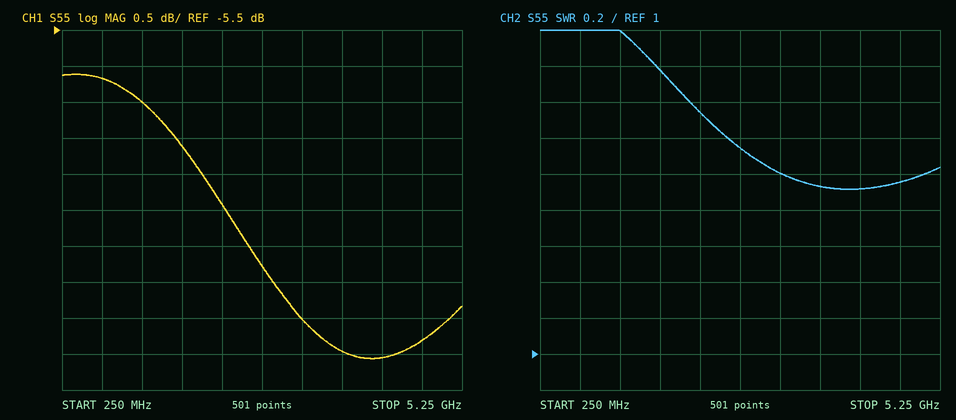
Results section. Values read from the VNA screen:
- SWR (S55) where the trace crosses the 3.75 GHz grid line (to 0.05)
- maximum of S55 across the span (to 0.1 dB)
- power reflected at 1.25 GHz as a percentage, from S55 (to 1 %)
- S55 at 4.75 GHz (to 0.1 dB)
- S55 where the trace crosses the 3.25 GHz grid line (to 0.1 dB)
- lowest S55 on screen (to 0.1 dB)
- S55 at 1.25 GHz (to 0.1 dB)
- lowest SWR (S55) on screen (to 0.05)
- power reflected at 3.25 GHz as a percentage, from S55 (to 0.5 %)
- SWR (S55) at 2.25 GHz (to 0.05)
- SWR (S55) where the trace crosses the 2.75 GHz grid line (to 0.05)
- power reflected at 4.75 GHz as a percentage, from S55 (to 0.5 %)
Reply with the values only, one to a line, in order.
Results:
1.95
-6.1 dB
22 %
-9.8 dB
-9.5 dB
-10.1 dB
-6.5 dB
1.90
11.0 %
2.35
2.15
10.5 %
